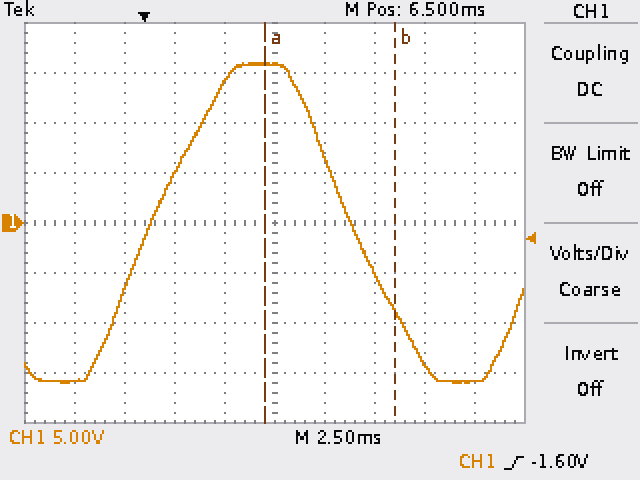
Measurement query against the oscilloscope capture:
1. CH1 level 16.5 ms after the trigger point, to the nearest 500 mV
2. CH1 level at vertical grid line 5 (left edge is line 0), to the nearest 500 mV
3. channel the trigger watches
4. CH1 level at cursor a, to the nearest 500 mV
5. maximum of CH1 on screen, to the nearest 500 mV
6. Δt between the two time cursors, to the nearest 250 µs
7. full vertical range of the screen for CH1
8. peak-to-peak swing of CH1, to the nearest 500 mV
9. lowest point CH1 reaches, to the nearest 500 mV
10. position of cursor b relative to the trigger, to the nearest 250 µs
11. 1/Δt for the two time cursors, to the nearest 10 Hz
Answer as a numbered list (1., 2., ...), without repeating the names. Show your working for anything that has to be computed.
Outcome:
1. -16.0 V
2. 16.0 V
3. CH1
4. 16.0 V
5. 16.0 V
6. 6.50 ms
7. 40 V
8. 16.0 V − (-16.0 V) = 32.0 V
9. -16.0 V
10. +12.50 ms
11. 1 / 6.50 ms ≈ 150 Hz
